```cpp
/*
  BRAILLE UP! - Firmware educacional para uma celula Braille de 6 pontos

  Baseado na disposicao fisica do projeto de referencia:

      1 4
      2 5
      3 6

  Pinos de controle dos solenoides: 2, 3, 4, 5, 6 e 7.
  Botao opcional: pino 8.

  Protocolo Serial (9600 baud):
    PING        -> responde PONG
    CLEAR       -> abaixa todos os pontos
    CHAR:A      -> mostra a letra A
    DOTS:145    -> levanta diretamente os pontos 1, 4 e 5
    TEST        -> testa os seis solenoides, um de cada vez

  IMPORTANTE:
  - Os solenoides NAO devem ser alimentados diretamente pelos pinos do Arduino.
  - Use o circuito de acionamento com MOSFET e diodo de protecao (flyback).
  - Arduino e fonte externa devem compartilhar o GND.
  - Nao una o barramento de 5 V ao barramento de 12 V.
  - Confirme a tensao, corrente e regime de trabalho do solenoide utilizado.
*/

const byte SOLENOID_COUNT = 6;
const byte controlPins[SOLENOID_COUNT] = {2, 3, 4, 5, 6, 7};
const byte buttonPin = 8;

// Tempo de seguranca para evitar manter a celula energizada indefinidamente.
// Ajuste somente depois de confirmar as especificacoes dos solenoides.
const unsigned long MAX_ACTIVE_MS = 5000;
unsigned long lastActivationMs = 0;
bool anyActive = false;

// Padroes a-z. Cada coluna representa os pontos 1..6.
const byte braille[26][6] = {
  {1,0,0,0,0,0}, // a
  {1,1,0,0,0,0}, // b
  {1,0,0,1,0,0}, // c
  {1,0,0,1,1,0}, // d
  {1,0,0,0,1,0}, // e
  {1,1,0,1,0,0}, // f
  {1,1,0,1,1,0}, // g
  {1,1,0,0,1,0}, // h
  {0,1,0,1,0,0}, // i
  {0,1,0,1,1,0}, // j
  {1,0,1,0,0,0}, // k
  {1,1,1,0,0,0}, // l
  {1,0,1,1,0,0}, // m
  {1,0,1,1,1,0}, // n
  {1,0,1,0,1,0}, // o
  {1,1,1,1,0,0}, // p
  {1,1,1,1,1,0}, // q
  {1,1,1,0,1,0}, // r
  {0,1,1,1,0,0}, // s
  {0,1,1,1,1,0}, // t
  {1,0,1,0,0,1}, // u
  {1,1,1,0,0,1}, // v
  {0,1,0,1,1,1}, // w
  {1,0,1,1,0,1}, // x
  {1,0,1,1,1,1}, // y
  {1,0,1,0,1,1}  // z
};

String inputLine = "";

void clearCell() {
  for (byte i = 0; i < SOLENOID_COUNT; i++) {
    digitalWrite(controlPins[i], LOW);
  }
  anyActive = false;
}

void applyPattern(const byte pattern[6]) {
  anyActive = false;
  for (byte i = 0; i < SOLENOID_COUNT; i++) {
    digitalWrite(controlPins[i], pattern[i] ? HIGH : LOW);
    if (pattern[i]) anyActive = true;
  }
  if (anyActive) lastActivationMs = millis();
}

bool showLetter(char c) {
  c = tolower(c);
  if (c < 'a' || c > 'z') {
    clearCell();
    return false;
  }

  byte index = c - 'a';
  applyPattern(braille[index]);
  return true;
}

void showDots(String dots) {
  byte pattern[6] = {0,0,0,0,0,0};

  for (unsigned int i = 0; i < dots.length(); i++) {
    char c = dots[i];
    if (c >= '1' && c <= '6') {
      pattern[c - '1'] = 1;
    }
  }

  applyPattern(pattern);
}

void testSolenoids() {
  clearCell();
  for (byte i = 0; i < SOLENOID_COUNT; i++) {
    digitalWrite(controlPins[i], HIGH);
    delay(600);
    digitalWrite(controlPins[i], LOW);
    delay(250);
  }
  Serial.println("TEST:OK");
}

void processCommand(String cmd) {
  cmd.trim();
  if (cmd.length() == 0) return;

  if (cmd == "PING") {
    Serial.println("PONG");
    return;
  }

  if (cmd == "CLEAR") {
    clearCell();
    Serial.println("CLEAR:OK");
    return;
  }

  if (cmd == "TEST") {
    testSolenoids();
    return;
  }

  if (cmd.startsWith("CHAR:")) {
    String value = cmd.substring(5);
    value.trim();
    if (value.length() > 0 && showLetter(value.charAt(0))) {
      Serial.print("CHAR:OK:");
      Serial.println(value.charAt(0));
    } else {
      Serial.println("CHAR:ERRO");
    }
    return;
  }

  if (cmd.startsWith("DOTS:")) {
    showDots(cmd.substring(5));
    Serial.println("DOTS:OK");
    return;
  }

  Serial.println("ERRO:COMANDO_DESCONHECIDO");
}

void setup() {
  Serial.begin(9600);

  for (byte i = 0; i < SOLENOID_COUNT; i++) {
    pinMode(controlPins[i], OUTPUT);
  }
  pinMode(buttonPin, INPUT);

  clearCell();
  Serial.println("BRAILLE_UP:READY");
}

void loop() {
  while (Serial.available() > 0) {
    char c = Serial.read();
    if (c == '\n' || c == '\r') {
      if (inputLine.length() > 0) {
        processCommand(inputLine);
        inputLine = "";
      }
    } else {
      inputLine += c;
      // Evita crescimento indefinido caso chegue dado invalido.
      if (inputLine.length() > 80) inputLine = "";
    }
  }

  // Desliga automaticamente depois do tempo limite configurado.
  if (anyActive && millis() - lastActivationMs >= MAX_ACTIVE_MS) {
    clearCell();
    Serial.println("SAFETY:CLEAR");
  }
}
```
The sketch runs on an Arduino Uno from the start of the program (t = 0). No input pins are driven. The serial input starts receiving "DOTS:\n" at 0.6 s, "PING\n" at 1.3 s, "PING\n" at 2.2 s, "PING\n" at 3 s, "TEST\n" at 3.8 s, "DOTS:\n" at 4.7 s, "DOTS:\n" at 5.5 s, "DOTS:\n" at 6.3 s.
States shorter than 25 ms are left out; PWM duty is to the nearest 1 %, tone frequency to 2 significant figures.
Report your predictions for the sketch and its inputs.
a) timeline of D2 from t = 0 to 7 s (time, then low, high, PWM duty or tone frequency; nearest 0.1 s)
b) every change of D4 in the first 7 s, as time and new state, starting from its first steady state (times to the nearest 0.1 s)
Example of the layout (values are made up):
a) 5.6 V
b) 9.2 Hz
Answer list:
a) 0 s low; 3.8 s high; 4.4 s low
b) 0 s low; 5.5 s high; 6.1 s low
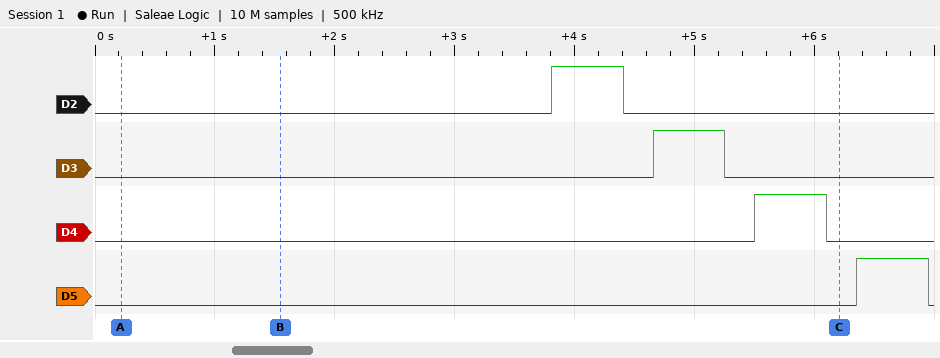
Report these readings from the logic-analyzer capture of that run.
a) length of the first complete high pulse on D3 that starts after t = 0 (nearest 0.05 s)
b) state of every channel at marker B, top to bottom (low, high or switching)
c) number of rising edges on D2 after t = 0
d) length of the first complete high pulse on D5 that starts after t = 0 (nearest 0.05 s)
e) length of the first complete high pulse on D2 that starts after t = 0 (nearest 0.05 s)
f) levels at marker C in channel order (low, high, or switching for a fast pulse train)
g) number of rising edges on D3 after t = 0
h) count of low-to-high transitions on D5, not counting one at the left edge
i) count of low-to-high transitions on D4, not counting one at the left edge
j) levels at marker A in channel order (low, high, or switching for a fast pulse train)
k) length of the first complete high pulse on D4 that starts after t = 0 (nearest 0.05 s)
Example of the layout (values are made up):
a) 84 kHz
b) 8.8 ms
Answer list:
a) 0.60 s
b) D2 low, D3 low, D4 low, D5 low
c) 1
d) 0.60 s
e) 0.60 s
f) D2 low, D3 low, D4 low, D5 low
g) 1
h) 1
i) 1
j) D2 low, D3 low, D4 low, D5 low
k) 0.60 s
